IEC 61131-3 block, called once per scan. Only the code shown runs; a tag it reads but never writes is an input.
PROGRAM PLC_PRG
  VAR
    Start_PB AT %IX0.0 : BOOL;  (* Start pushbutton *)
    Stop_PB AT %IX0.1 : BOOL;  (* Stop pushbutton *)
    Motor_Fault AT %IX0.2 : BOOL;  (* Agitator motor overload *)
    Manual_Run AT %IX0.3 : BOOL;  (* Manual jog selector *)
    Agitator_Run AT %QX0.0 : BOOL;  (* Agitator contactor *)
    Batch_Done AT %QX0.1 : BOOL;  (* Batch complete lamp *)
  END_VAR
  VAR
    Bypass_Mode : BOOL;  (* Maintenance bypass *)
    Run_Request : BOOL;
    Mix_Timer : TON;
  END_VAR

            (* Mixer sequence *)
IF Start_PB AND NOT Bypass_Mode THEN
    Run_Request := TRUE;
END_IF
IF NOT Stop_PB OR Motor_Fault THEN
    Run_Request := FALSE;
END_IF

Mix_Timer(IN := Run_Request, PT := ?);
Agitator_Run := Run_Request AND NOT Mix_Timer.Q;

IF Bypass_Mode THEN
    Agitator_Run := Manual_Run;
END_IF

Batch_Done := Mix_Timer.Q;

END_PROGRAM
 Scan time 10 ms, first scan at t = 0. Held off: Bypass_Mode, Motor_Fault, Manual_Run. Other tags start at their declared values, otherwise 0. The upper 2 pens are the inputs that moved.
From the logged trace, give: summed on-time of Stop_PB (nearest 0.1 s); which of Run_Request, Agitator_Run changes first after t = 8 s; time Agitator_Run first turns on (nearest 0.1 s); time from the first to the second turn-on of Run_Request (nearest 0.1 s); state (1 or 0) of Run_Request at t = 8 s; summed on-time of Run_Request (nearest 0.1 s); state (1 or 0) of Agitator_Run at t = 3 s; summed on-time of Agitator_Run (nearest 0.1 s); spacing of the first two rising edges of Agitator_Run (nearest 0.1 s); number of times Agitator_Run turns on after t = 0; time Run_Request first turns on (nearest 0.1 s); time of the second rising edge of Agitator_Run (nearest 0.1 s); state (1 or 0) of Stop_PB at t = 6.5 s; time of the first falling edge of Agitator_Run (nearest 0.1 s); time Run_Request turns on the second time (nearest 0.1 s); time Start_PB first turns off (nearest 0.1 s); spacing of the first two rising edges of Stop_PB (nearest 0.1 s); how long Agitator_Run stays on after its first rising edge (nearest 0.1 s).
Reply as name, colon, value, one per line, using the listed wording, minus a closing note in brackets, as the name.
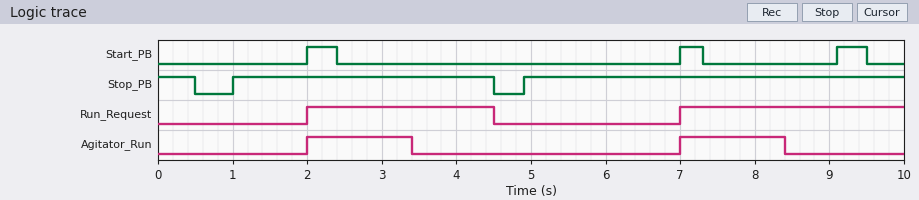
summed on-time of Stop_PB: 9.1 s
which of Run_Request, Agitator_Run changes first after t = 8 s: Agitator_Run
time Agitator_Run first turns on: 2.0 s
time from the first to the second turn-on of Run_Request: 5.0 s
state (1 or 0) of Run_Request at t = 8 s: 1
summed on-time of Run_Request: 5.5 s
state (1 or 0) of Agitator_Run at t = 3 s: 1
summed on-time of Agitator_Run: 2.8 s
spacing of the first two rising edges of Agitator_Run: 5.0 s
number of times Agitator_Run turns on after t = 0: 2
time Run_Request first turns on: 2.0 s
time of the second rising edge of Agitator_Run: 7.0 s
state (1 or 0) of Stop_PB at t = 6.5 s: 1
time of the first falling edge of Agitator_Run: 3.4 s
time Run_Request turns on the second time: 7.0 s
time Start_PB first turns off: 2.4 s
spacing of the first two rising edges of Stop_PB: 3.9 s
how long Agitator_Run stays on after its first rising edge: 1.4 s
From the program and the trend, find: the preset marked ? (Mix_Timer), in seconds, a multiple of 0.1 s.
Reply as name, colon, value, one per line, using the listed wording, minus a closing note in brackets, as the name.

the preset marked ? (Mix_Timer), in seconds, a multiple of 0.1 s: 1.4 s
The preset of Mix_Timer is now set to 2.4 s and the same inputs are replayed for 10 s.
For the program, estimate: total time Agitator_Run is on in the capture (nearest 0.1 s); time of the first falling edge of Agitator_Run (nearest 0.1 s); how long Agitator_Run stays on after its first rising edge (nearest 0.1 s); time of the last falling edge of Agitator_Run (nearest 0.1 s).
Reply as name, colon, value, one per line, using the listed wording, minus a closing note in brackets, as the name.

total time Agitator_Run is on in the capture: 4.8 s
time of the first falling edge of Agitator_Run: 4.4 s
how long Agitator_Run stays on after its first rising edge: 2.4 s
time of the last falling edge of Agitator_Run: 9.4 s
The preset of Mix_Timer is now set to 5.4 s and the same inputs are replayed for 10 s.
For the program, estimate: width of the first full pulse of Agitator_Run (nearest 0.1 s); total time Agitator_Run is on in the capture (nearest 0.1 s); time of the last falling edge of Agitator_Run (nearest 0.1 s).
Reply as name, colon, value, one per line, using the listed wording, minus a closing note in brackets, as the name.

width of the first full pulse of Agitator_Run: 2.5 s
total time Agitator_Run is on in the capture: 5.5 s
time of the last falling edge of Agitator_Run: 4.5 s
